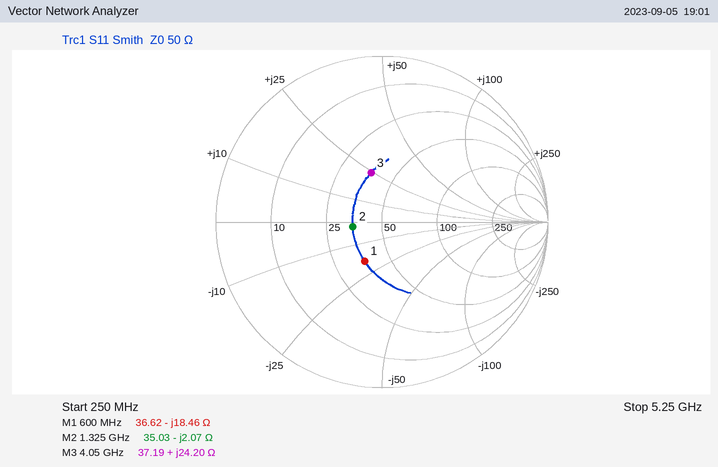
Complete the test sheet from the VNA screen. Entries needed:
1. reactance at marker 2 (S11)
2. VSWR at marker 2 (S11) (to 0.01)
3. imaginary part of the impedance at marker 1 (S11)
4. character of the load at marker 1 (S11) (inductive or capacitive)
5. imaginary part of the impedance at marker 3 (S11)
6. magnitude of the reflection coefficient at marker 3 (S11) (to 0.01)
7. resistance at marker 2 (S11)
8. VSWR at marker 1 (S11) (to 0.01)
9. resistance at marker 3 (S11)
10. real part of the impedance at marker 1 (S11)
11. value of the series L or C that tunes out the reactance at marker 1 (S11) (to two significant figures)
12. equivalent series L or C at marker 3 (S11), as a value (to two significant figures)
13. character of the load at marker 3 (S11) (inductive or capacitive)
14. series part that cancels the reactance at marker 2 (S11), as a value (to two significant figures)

-2.07 Ω
1.43
-18.46 Ω
capacitive
+24.20 Ω
0.30
35.03 Ω
1.69
37.19 Ω
36.62 Ω
4.9 nH
950 pH
inductive
250 pH
